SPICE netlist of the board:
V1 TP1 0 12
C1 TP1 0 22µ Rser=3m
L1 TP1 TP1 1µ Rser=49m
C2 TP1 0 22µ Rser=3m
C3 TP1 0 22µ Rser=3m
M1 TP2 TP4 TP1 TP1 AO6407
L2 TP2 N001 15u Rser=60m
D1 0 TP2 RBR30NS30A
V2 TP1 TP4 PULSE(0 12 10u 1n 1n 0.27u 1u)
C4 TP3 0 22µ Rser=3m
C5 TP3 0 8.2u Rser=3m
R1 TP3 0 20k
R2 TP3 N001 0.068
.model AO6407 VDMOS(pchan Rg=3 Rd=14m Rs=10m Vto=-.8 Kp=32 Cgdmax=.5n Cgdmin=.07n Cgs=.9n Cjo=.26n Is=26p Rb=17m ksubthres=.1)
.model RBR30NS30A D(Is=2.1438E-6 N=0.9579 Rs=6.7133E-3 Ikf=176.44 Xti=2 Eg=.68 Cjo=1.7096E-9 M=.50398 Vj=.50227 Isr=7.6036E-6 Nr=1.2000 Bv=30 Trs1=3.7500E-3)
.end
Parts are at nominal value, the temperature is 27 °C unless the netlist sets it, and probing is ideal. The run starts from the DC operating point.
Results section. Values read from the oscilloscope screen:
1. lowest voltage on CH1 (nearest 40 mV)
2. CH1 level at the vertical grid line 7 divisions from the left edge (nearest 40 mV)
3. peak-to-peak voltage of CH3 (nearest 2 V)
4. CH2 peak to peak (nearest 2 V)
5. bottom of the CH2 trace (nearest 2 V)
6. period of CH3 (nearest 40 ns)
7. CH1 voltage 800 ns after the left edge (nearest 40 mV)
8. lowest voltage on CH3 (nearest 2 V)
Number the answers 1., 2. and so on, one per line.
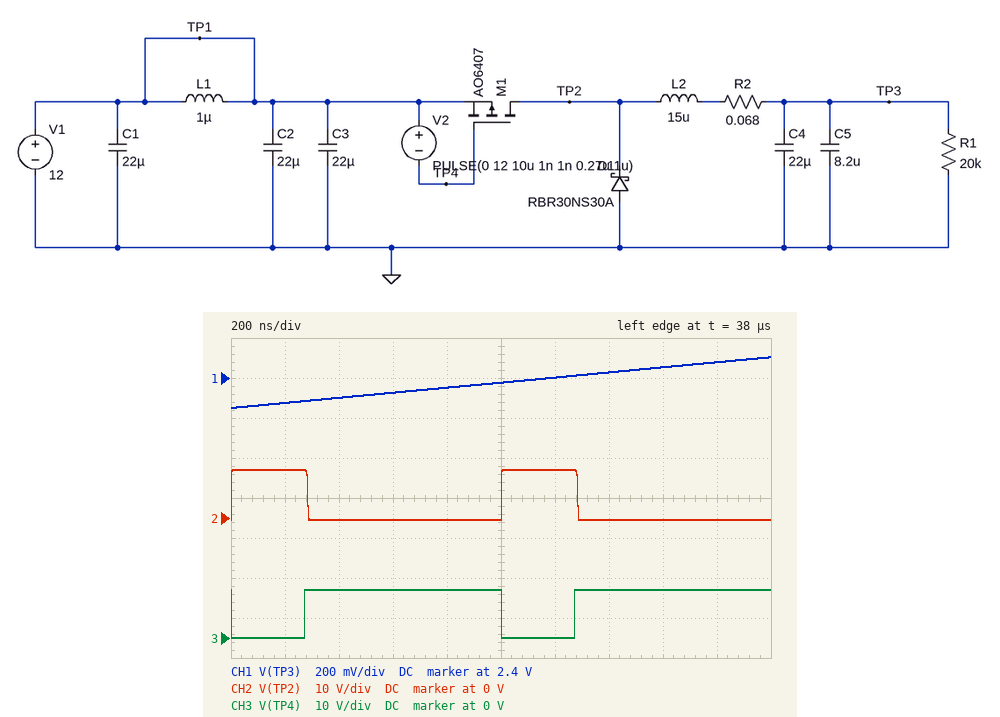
1. 2.24 V
2. 2.44 V
3. 12 V
4. 12 V
5. 0 V
6. 1.00 µs
7. 2.36 V
8. 0 V
